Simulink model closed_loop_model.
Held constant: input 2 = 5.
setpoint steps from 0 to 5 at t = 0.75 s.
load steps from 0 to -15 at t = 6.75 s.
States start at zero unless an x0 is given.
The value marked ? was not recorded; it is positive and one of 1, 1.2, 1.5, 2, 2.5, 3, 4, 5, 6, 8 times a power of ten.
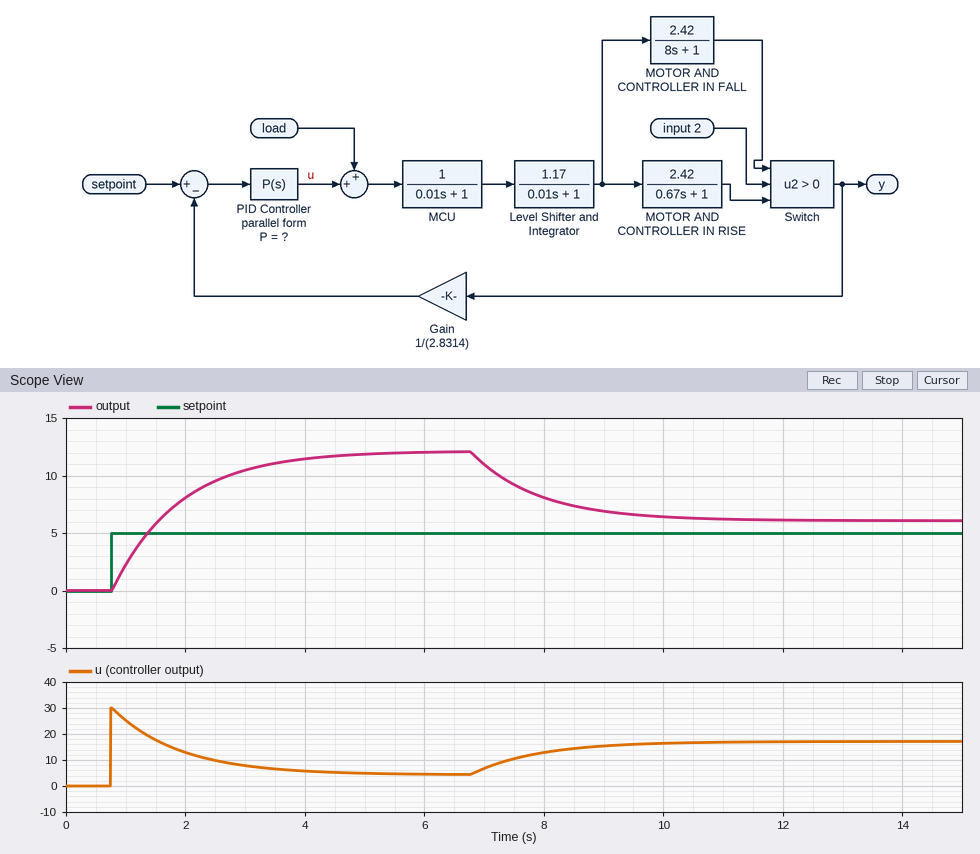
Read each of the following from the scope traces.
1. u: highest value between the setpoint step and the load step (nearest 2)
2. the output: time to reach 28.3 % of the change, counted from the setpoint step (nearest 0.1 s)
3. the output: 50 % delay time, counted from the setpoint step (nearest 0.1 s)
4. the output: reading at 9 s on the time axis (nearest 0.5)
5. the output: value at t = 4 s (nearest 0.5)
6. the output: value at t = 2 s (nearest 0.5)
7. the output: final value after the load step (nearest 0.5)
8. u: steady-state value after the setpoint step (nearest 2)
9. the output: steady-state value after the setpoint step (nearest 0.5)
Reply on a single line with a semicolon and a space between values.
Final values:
30; 0.4 s; 0.8 s; 7.0; 11.5; 8.0; 6.0; 4; 12.0
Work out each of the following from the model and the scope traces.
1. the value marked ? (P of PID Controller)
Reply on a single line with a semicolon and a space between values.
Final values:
6
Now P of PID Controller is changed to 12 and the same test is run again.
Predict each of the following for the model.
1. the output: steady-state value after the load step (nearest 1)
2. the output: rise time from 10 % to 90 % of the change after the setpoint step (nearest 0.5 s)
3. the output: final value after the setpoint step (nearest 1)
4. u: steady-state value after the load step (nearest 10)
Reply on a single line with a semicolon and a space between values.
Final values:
10; 1.5 s; 13; 20
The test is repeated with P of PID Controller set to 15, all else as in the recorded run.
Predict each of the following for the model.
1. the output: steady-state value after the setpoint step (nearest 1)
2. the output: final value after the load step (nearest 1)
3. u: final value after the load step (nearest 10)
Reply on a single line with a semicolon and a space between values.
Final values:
13; 11; 20
